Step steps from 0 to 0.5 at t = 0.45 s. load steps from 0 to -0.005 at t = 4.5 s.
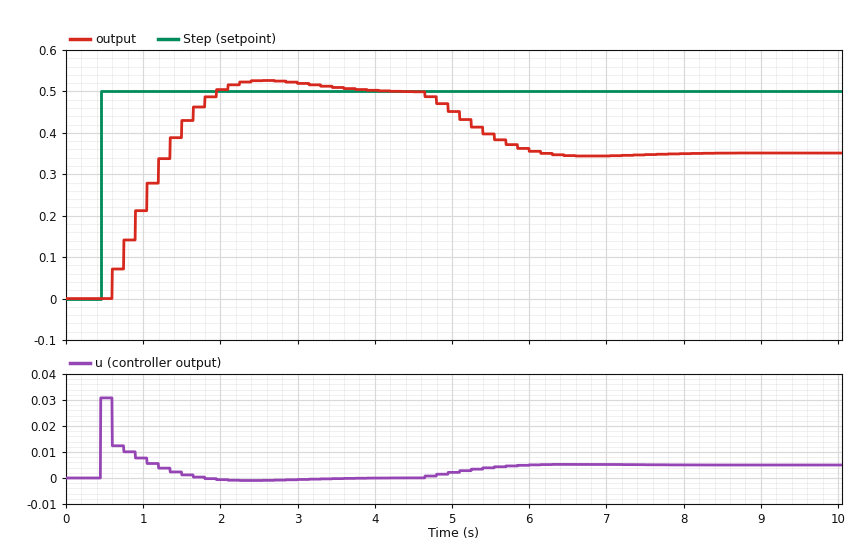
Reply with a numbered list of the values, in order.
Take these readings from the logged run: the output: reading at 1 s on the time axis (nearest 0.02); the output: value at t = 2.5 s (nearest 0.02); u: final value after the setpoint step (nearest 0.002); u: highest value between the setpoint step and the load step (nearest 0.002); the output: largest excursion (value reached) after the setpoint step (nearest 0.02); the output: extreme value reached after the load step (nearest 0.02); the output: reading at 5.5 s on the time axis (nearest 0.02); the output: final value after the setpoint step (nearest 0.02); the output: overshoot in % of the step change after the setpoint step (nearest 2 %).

1. 0.22
2. 0.52
3. 0.000
4. 0.030
5. 0.52
6. 0.34
7. 0.40
8. 0.50
9. 6 %
